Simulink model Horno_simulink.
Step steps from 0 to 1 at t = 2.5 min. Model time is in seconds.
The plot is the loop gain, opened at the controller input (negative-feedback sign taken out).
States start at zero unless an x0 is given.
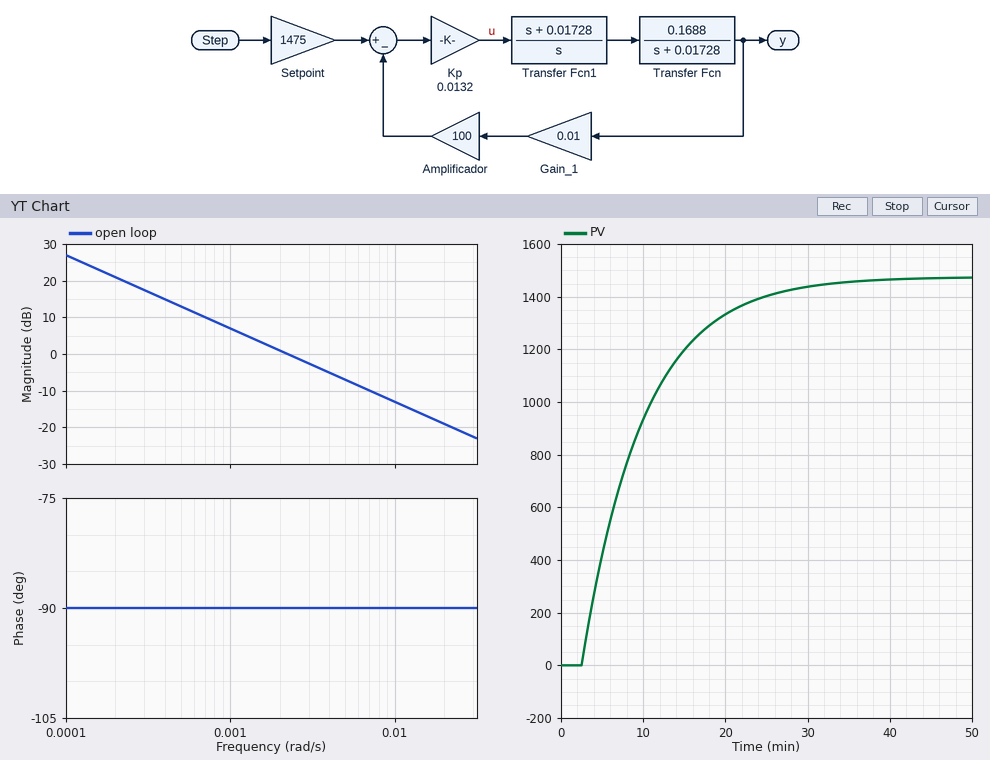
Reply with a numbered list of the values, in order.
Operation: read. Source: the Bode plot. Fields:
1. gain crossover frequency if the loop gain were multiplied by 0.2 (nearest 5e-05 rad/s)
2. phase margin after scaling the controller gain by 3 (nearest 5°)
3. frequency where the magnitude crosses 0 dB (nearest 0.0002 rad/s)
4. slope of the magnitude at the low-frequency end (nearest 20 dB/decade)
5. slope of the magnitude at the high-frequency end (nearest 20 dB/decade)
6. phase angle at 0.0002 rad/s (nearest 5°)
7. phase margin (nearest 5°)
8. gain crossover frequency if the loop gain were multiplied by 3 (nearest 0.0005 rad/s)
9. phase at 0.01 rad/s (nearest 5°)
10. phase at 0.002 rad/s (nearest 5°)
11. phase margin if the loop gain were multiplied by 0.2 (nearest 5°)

1. 0.00045 rad/s
2. 90°
3. 0.0022 rad/s
4. -20 dB/decade
5. -20 dB/decade
6. -90°
7. 90°
8. 0.0065 rad/s
9. -90°
10. -90°
11. 90°
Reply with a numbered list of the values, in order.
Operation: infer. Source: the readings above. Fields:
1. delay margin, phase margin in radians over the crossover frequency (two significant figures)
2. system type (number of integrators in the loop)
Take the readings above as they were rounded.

1. 710 s
2. 1
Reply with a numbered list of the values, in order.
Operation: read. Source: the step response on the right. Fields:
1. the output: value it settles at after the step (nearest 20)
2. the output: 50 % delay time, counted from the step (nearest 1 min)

1. 1480
2. 5 min
